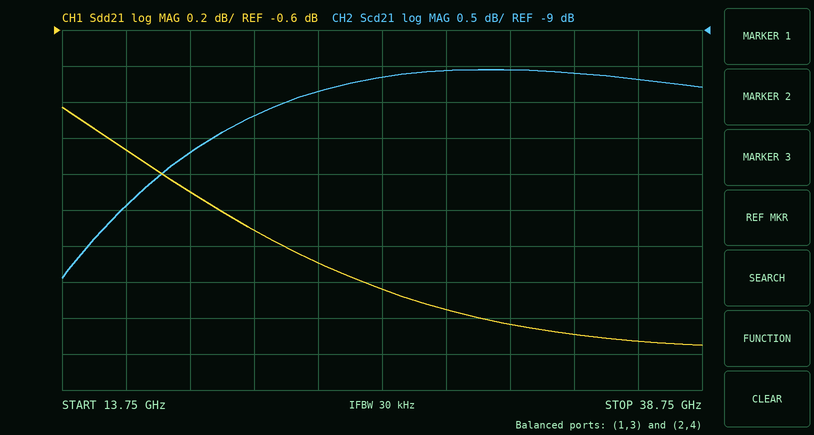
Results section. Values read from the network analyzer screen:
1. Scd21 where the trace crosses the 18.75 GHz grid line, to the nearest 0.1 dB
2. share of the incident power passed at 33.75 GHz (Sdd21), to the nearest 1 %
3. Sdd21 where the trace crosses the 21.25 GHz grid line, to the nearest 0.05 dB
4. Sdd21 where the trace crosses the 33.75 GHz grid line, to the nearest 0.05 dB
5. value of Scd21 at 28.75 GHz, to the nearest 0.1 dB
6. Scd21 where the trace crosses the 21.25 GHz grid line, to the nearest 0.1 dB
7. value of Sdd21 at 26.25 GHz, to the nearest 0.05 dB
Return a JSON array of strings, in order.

["-10.7 dB", "59 %", "-1.70 dB", "-2.30 dB", "-9.6 dB", "-10.2 dB", "-2.05 dB"]
